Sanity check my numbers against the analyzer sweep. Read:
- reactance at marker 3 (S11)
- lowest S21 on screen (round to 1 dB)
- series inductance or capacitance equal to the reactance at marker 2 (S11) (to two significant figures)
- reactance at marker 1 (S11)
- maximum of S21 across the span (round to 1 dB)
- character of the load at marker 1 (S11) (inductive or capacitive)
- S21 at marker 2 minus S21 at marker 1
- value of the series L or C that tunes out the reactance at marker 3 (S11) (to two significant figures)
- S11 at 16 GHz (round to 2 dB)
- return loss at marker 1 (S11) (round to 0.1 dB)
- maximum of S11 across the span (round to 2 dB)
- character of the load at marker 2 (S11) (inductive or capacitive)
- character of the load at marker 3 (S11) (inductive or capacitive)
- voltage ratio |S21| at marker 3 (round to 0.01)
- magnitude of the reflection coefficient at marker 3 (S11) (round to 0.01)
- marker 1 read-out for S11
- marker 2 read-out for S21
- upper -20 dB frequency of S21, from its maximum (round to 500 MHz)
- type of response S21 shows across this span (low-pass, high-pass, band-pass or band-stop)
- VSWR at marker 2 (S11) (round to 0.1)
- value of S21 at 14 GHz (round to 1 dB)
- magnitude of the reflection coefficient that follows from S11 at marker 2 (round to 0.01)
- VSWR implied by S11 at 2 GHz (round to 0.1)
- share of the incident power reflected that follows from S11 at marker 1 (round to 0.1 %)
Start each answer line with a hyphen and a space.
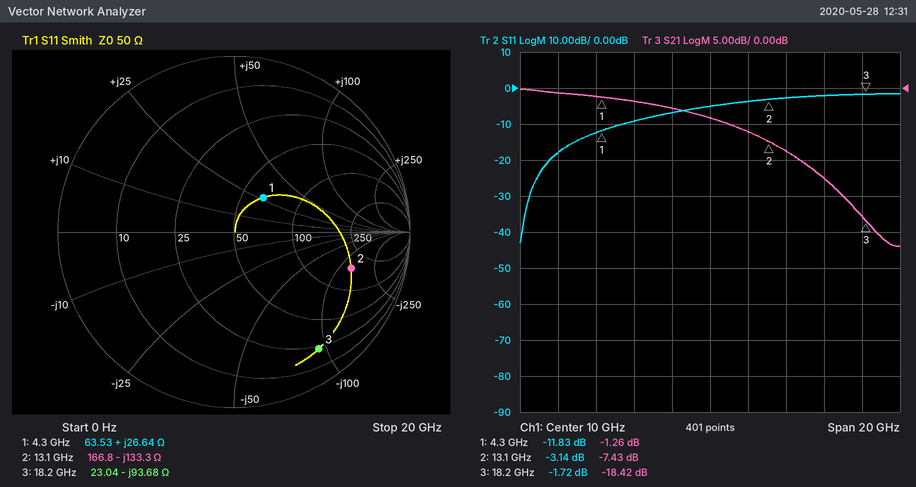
- -93.68 Ω
- -22 dB
- 91 fF
- +26.64 Ω
- 0 dB
- inductive
- -6.17 dB
- 820 pH
- -2 dB
- 11.8 dB
- -2 dB
- capacitive
- capacitive
- 0.12
- 0.82
- -11.83 dB
- -7.43 dB
- 19.0 GHz
- low-pass
- 5.6
- -9 dB
- 0.70
- 1.3
- 6.6 %
